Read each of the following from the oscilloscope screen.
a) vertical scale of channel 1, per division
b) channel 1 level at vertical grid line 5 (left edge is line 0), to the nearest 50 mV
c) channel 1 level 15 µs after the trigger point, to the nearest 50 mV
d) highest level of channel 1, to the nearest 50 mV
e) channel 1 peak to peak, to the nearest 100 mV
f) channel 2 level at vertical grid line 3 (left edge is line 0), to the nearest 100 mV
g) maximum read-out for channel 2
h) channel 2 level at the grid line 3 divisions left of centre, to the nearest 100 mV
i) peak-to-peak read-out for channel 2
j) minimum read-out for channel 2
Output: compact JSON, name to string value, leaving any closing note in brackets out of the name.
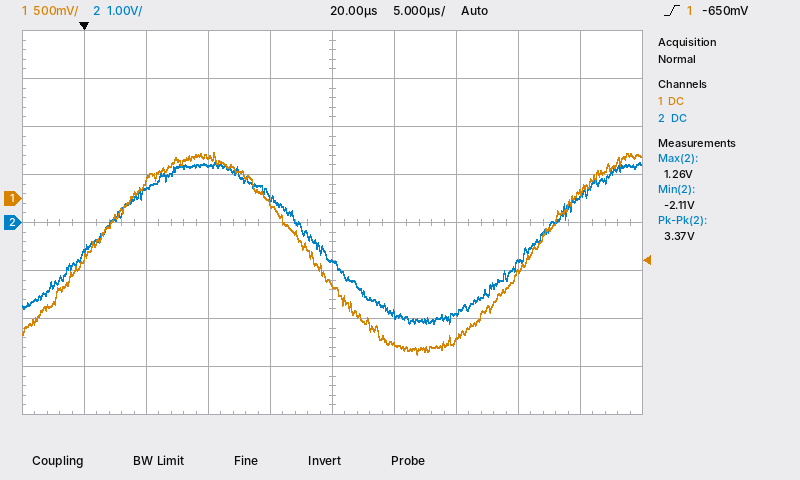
{"vertical scale of channel 1, per division": "500 mV", "channel 1 level at vertical grid line 5 (left edge is line 0), to the nearest 50 mV": "-900 mV", "channel 1 level 15 µs after the trigger point, to the nearest 50 mV": "-50 mV", "highest level of channel 1, to the nearest 50 mV": "500 mV", "channel 1 peak to peak, to the nearest 100 mV": "2.10 V", "channel 2 level at vertical grid line 3 (left edge is line 0), to the nearest 100 mV": "1.2 V", "maximum read-out for channel 2": "1.26 V", "channel 2 level at the grid line 3 divisions left of centre, to the nearest 100 mV": "700 mV", "peak-to-peak read-out for channel 2": "3.37 V", "minimum read-out for channel 2": "-2.11 V"}
